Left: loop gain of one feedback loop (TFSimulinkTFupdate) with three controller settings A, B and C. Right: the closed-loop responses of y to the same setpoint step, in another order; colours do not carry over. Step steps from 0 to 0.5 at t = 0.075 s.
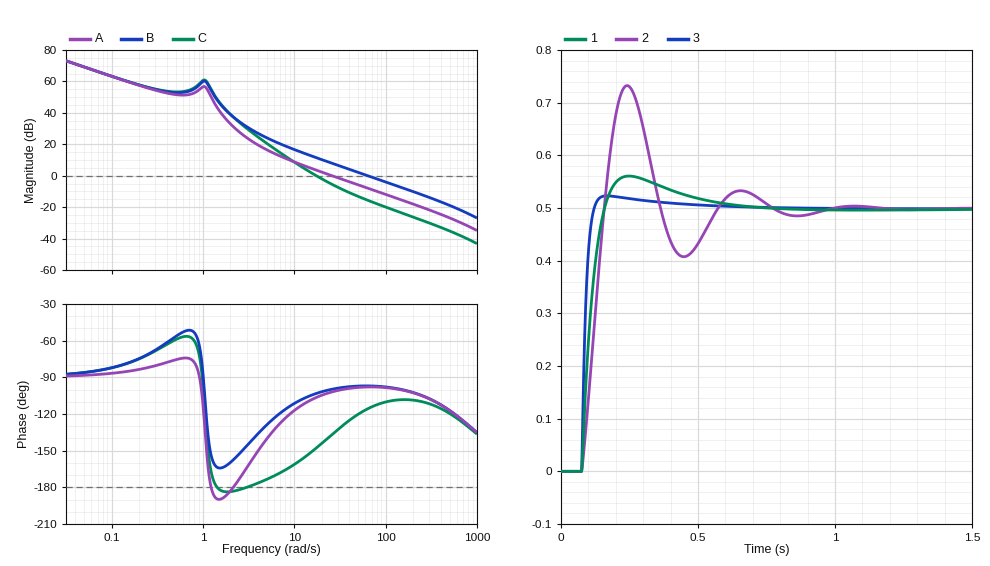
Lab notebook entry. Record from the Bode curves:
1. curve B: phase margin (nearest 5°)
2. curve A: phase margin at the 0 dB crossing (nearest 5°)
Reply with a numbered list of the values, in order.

1. 85°
2. 80°
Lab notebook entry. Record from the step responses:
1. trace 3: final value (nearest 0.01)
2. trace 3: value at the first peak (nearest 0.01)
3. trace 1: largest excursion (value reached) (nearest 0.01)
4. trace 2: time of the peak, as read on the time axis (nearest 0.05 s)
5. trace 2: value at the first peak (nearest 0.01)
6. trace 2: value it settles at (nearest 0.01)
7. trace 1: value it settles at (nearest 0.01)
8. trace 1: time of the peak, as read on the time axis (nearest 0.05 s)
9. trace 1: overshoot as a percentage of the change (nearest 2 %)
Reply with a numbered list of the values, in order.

1. 0.50
2. 0.52
3. 0.56
4. 0.25 s
5. 0.73
6. 0.50
7. 0.50
8. 0.25 s
9. 12 %
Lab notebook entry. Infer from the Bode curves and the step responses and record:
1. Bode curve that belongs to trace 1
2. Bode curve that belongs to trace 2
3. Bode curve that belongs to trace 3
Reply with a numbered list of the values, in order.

1. A
2. C
3. B
